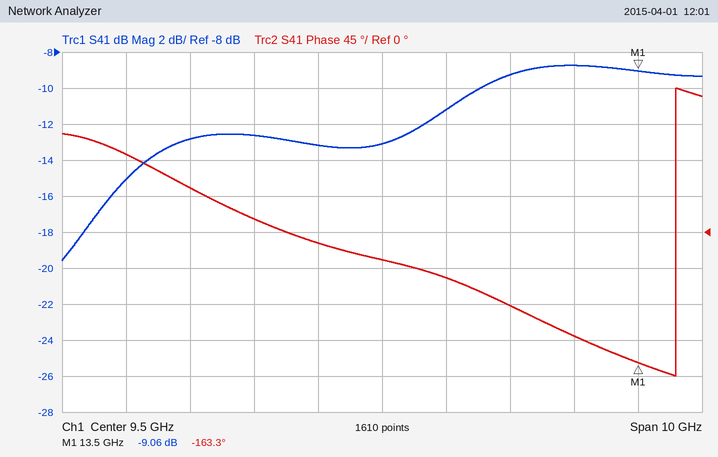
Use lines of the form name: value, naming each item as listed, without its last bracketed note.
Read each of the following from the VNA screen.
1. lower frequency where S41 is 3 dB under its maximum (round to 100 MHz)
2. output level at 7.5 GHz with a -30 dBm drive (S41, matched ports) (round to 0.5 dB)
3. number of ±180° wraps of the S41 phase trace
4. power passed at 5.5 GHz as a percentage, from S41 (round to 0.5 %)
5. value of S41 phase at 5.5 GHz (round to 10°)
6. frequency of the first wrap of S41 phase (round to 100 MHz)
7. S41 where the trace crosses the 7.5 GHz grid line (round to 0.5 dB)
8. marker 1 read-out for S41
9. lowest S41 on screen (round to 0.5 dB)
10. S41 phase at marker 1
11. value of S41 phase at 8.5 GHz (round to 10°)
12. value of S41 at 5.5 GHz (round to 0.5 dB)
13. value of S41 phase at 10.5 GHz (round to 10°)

lower frequency where S41 is 3 dB under its maximum: 10.3 GHz
output level at 7.5 GHz with a -30 dBm drive (S41, matched ports): -42.5 dBm
number of ±180° wraps of the S41 phase trace: 1
power passed at 5.5 GHz as a percentage, from S41: 3.0 %
value of S41 phase at 5.5 GHz: 100°
frequency of the first wrap of S41 phase: 14.1 GHz
S41 where the trace crosses the 7.5 GHz grid line: -12.5 dB
marker 1 read-out for S41: -9.06 dB
lowest S41 on screen: -19.5 dB
S41 phase at marker 1: -163.3°
value of S41 phase at 8.5 GHz: -10°
value of S41 at 5.5 GHz: -15.0 dB
value of S41 phase at 10.5 GHz: -60°
